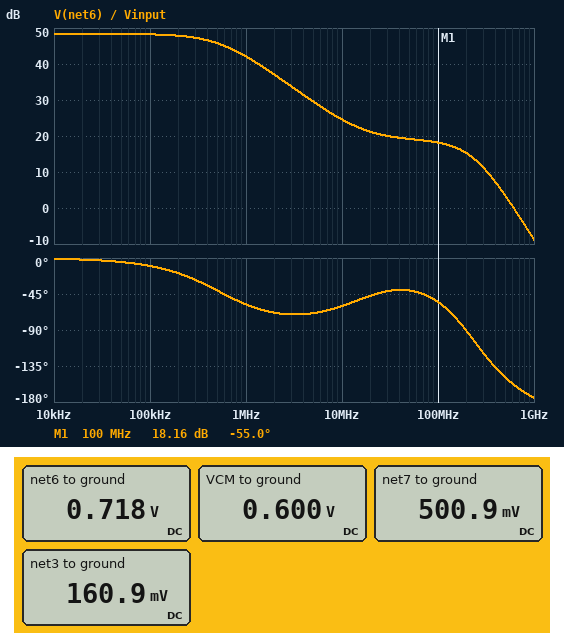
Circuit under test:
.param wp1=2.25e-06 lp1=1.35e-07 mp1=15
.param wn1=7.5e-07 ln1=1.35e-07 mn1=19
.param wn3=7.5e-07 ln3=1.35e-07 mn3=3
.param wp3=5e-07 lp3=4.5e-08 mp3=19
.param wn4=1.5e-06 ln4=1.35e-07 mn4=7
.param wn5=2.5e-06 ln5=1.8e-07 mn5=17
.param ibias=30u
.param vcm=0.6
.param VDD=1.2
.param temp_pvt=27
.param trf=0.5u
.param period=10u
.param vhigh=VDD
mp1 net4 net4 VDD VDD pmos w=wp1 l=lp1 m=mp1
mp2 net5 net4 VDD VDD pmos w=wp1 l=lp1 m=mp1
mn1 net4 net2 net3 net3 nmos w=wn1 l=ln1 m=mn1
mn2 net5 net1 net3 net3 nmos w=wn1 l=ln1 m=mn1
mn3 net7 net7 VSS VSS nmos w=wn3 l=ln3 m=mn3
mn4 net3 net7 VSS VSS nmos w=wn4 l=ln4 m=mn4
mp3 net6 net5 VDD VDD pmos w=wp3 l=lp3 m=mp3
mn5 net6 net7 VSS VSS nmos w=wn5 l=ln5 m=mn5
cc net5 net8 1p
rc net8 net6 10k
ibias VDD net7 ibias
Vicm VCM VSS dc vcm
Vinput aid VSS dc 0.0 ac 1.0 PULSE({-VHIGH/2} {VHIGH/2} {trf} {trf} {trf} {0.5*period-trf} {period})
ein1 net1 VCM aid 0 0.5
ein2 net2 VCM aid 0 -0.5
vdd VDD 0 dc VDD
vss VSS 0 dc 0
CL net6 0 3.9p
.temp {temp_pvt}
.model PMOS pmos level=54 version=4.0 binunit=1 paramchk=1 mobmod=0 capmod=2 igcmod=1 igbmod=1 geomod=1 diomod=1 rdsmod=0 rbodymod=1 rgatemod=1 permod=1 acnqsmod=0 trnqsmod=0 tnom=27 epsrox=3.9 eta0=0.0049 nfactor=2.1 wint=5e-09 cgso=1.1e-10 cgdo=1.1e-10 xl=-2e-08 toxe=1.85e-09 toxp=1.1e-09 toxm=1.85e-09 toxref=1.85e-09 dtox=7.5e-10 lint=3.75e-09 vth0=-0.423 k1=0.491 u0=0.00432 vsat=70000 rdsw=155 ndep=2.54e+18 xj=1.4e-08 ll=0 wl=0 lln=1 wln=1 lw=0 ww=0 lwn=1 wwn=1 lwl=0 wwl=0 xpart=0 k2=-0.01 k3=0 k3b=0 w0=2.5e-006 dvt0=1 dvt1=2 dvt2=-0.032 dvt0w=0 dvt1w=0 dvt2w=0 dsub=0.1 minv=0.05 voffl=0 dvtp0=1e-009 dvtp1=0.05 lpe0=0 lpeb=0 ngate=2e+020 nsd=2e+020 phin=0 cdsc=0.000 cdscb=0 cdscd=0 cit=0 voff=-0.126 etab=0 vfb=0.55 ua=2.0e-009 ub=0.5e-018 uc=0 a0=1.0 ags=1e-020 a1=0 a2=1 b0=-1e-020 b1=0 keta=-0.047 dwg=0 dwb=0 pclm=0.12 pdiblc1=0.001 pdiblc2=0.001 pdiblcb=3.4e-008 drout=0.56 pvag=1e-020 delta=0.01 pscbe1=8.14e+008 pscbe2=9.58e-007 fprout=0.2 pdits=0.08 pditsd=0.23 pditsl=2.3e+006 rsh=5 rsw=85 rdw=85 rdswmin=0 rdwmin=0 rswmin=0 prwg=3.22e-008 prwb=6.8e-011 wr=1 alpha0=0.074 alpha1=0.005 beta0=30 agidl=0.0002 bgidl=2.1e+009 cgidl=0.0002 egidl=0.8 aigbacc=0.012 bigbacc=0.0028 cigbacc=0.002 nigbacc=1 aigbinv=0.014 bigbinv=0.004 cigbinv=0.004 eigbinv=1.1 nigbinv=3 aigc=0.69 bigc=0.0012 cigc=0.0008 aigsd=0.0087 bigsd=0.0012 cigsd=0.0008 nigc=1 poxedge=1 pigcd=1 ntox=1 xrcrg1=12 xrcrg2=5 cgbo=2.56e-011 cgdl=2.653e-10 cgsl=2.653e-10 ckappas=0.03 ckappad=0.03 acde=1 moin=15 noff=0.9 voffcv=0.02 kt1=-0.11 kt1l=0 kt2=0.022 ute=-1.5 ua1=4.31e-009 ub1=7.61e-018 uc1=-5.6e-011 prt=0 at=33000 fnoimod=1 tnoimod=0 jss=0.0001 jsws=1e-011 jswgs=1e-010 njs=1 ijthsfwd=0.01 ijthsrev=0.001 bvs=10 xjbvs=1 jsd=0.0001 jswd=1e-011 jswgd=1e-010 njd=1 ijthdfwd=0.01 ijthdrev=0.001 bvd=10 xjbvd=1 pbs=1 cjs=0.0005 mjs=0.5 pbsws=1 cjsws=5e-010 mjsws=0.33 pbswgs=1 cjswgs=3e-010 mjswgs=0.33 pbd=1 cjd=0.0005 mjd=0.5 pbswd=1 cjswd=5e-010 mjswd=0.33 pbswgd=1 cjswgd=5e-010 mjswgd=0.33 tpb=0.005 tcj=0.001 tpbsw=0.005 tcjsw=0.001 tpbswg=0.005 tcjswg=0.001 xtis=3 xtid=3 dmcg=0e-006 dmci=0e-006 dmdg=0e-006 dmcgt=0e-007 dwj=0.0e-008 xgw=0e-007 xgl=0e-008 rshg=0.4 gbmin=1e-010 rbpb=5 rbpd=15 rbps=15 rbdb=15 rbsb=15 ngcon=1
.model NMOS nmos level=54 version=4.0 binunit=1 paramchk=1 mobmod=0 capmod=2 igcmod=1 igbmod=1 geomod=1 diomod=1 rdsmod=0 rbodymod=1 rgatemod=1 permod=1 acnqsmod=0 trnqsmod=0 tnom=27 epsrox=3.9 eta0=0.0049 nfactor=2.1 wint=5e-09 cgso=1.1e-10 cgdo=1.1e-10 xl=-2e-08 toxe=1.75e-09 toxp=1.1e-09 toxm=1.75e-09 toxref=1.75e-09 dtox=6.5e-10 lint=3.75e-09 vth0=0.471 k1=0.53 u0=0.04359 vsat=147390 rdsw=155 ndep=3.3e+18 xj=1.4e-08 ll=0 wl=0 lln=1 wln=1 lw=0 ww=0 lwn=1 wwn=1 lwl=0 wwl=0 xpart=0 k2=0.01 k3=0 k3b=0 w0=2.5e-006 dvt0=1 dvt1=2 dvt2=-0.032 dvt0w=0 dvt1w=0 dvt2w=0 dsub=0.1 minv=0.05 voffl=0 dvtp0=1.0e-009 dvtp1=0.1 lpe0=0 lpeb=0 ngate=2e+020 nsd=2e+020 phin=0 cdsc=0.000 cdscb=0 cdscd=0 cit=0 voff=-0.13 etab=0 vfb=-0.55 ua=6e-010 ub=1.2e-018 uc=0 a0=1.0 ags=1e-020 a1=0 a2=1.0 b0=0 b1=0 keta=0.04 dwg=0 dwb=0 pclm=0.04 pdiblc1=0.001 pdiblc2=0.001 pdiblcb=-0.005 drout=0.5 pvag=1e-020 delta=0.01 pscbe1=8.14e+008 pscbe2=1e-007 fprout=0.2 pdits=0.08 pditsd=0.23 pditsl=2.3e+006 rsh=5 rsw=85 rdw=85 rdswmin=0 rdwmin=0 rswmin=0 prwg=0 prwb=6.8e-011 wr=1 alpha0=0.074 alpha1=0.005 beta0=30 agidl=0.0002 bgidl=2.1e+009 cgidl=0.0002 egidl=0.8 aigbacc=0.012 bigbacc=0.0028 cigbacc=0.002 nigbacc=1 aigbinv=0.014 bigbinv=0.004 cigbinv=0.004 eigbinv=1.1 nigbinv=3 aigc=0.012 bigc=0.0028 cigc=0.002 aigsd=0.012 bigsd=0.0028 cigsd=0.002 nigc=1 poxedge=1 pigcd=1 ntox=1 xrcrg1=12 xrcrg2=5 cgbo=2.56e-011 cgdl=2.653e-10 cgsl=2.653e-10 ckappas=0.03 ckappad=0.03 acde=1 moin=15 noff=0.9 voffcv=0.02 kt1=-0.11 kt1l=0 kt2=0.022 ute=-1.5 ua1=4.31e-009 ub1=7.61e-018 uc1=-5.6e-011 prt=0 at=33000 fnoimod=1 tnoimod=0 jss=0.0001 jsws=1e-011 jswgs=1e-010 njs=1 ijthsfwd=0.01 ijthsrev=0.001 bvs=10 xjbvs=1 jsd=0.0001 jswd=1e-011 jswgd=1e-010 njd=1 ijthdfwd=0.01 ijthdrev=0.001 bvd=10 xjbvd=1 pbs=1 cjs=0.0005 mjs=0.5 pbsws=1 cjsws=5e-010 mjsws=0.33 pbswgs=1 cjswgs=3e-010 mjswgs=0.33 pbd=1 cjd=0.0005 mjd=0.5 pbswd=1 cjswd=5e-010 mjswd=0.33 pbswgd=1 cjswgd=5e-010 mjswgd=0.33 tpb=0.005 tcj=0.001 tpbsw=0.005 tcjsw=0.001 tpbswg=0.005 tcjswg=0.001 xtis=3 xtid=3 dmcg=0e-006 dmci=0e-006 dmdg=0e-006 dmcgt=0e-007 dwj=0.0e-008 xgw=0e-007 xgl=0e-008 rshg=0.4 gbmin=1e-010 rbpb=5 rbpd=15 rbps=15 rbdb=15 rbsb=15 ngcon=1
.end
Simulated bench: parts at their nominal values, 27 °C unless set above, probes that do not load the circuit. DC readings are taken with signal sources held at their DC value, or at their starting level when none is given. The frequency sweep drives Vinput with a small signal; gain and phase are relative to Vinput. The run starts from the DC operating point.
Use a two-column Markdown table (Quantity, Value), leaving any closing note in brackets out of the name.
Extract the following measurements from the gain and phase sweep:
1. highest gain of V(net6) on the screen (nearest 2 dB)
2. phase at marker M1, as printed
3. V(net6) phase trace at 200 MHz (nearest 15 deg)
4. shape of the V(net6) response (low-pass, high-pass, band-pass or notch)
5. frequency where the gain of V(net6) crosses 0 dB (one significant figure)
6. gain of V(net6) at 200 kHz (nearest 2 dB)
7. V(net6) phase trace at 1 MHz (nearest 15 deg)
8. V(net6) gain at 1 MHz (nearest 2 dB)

| Quantity | Value |
|---|---|
| highest gain of V(net6) on the screen | 48 dB |
| phase at marker M1, as printed | -55.0 deg |
| V(net6) phase trace at 200 MHz | -90 deg |
| shape of the V(net6) response | low-pass |
| frequency where the gain of V(net6) crosses 0 dB | 600 MHz |
| gain of V(net6) at 200 kHz | 48 dB |
| V(net6) phase trace at 1 MHz | -60 deg |
| V(net6) gain at 1 MHz | 42 dB |
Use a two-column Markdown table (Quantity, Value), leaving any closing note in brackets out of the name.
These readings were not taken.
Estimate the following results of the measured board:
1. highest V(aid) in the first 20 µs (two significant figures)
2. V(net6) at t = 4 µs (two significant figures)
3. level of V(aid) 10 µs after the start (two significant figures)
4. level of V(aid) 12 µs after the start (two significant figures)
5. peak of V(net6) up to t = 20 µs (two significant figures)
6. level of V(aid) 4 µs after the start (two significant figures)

| Quantity | Value |
|---|---|
| highest V(aid) in the first 20 µs | 600 mV |
| V(net6) at t = 4 µs | 1.2 V |
| level of V(aid) 10 µs after the start | -600 mV |
| level of V(aid) 12 µs after the start | 600 mV |
| peak of V(net6) up to t = 20 µs | 1.2 V |
| level of V(aid) 4 µs after the start | 600 mV |
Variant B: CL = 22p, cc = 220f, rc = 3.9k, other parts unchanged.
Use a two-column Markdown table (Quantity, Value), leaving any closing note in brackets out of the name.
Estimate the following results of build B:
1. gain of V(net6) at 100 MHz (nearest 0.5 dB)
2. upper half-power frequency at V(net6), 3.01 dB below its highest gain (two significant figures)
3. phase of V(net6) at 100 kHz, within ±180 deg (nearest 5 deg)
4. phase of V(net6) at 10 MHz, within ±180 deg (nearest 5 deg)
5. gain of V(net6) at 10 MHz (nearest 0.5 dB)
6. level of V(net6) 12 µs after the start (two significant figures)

| Quantity | Value |
|---|---|
| gain of V(net6) at 100 MHz | 5.5 dB |
| upper half-power frequency at V(net6), 3.01 dB below its highest gain | 1.9 MHz |
| phase of V(net6) at 100 kHz, within ±180 deg | -5 deg |
| phase of V(net6) at 10 MHz, within ±180 deg | -95 deg |
| gain of V(net6) at 10 MHz | 33.5 dB |
| level of V(net6) 12 µs after the start | 1.2 V |
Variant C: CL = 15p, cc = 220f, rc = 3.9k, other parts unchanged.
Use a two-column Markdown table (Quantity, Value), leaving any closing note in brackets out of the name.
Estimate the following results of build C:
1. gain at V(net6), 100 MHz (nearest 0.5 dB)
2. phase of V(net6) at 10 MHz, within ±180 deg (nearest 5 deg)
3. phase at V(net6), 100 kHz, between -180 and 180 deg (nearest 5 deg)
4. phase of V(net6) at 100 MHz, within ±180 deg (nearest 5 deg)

| Quantity | Value |
|---|---|
| gain at V(net6), 100 MHz | 8.5 dB |
| phase of V(net6) at 10 MHz, within ±180 deg | -90 deg |
| phase at V(net6), 100 kHz, between -180 and 180 deg | -5 deg |
| phase of V(net6) at 100 MHz, within ±180 deg | -135 deg |
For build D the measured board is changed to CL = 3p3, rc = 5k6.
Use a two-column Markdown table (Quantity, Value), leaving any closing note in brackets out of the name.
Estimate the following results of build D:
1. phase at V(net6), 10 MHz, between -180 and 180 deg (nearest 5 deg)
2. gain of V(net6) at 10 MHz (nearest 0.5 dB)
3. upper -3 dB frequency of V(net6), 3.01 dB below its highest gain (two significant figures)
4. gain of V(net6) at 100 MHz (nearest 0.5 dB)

| Quantity | Value |
|---|---|
| phase at V(net6), 10 MHz, between -180 and 180 deg | -70 deg |
| gain of V(net6) at 10 MHz | 24.0 dB |
| upper -3 dB frequency of V(net6), 3.01 dB below its highest gain | 560 kHz |
| gain of V(net6) at 100 MHz | 13.5 dB |
